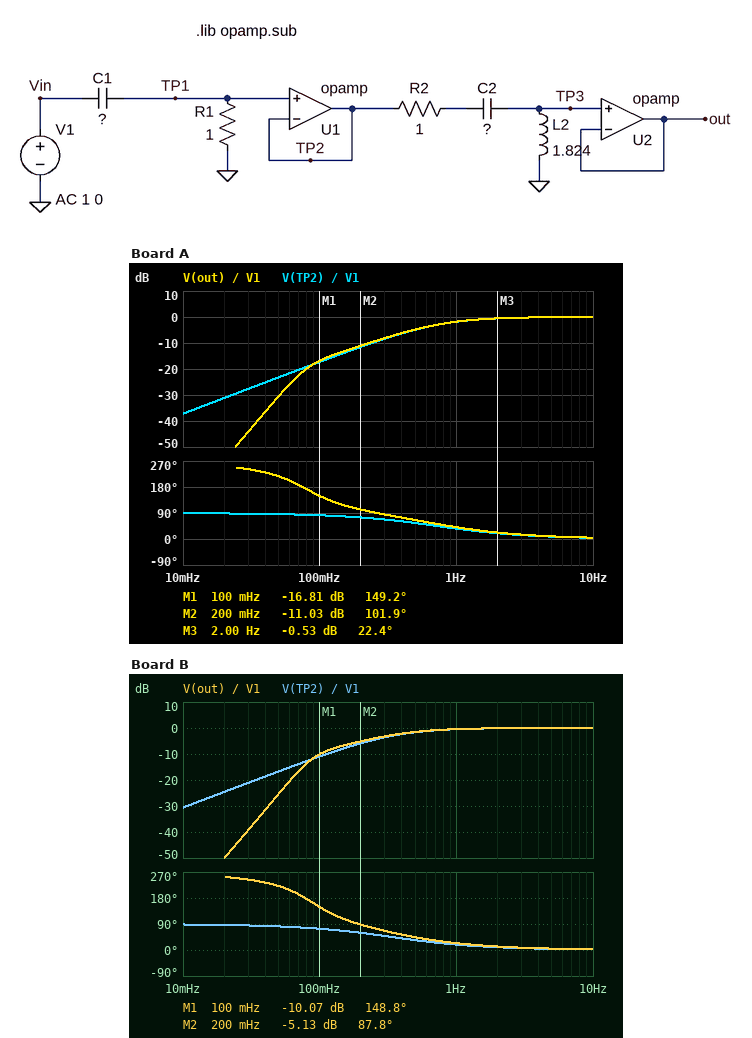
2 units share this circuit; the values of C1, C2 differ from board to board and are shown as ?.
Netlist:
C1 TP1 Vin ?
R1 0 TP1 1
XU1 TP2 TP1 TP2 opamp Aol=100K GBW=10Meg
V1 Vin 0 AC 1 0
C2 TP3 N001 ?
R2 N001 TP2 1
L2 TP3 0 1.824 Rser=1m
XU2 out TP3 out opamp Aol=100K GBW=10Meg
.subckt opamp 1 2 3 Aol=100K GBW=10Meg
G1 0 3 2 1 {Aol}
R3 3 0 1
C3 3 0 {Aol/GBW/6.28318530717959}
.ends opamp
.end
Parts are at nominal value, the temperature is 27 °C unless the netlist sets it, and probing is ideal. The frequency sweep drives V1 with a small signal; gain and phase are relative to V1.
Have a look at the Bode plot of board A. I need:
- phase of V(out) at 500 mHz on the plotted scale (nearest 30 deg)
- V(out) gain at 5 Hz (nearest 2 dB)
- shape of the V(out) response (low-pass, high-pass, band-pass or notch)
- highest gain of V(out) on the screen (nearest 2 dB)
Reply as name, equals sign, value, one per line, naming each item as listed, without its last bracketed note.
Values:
phase of V(out) at 500 mHz on the plotted scale = 60 deg
V(out) gain at 5 Hz = 0 dB
shape of the V(out) response = high-pass
highest gain of V(out) on the screen = 0 dB
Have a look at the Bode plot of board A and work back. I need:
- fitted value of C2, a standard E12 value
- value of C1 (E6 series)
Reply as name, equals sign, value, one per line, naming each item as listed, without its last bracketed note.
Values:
fitted value of C2, a standard E12 value = 2.2 F
value of C1 = 220 mF
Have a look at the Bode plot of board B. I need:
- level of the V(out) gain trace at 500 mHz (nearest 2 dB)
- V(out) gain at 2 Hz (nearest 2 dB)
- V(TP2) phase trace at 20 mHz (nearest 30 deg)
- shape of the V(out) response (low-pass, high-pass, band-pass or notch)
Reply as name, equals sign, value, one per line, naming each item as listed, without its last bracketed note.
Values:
level of the V(out) gain trace at 500 mHz = -2 dB
V(out) gain at 2 Hz = 0 dB
V(TP2) phase trace at 20 mHz = 90 deg
shape of the V(out) response = high-pass
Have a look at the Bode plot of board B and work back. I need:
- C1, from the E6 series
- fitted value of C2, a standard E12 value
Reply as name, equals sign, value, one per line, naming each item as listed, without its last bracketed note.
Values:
C1, from the E6 series = 470 mF
fitted value of C2, a standard E12 value = 1.8 F
